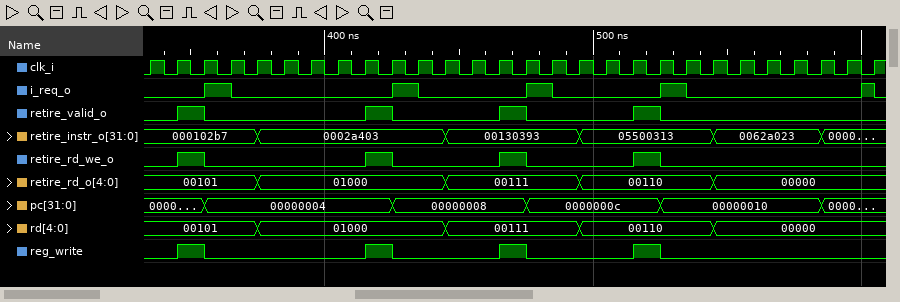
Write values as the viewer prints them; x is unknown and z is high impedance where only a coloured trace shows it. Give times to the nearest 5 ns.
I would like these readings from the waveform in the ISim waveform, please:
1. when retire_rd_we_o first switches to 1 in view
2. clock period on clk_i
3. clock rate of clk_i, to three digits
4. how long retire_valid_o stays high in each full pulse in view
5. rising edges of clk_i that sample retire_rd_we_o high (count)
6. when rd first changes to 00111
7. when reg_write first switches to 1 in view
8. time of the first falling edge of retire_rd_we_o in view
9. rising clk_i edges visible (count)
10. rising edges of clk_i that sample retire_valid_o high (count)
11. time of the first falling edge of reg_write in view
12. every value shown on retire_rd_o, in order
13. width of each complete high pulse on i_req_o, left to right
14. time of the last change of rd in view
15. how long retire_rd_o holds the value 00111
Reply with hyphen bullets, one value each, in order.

- 345 ns
- 10 ns
- 100 MHz
- 10 ns, 10 ns, 10 ns, 10 ns
- 4
- 445 ns
- 345 ns
- 355 ns
- 28
- 4
- 355 ns
- 00101, 01000, 00111, 00110, 00000
- 10 ns, 10 ns, 10 ns, 10 ns, 5 ns
- 545 ns
- 50 ns
